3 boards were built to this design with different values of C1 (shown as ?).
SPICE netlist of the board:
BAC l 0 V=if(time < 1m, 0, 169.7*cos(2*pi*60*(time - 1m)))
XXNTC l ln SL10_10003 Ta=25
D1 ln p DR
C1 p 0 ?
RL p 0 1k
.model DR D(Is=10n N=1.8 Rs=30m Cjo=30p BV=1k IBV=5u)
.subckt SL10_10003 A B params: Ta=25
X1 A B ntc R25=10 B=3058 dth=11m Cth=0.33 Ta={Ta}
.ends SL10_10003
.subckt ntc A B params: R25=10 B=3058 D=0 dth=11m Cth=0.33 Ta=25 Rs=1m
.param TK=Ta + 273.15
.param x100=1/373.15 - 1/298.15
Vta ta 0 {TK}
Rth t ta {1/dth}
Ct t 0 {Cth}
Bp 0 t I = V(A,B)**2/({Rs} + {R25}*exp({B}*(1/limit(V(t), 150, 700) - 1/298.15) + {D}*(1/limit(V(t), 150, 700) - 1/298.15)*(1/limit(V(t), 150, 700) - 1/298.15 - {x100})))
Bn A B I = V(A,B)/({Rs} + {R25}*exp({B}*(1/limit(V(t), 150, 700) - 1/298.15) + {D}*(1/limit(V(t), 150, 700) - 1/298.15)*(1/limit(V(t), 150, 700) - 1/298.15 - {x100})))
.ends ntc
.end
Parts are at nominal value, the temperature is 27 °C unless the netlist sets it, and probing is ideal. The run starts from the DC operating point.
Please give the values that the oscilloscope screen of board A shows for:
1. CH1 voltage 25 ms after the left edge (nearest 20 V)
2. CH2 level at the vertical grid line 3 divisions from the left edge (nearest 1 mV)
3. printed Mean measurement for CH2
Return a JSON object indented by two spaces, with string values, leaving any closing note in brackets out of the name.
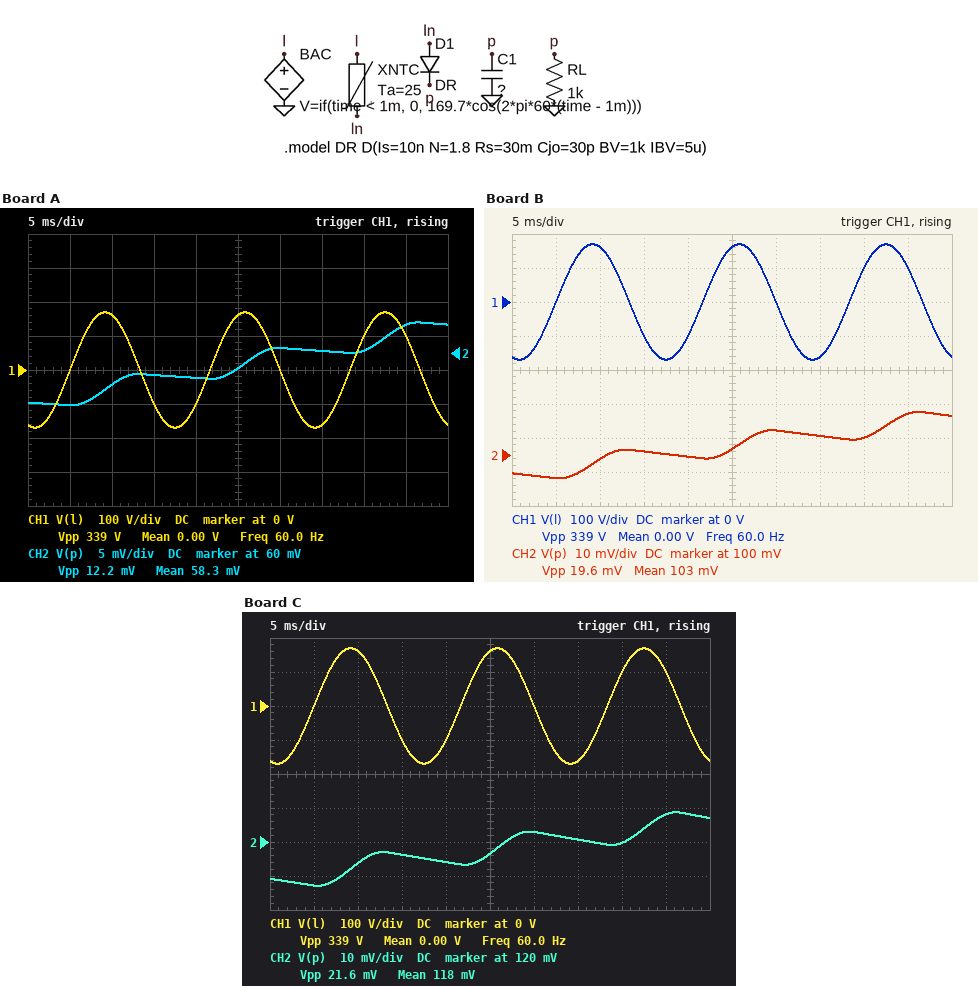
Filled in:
{
  "CH1 voltage 25 ms after the left edge": "160 V",
  "CH2 level at the vertical grid line 3 divisions from the left edge": "57 mV",
  "printed Mean measurement for CH2": "58.3 mV"
}
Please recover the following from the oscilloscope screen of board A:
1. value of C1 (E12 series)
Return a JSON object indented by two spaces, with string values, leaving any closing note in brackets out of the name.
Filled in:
{
  "value of C1": "680 µF"
}
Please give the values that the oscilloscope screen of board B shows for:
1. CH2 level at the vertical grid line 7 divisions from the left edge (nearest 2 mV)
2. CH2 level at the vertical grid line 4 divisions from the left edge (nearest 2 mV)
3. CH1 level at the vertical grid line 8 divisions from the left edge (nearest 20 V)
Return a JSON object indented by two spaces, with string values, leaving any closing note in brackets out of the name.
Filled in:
{
  "CH2 level at the vertical grid line 7 divisions from the left edge": "106 mV",
  "CH2 level at the vertical grid line 4 divisions from the left edge": "100 mV",
  "CH1 level at the vertical grid line 8 divisions from the left edge": "100 V"
}
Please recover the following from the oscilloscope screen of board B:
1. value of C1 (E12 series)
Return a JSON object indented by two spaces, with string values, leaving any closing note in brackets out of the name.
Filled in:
{
  "value of C1": "330 µF"
}
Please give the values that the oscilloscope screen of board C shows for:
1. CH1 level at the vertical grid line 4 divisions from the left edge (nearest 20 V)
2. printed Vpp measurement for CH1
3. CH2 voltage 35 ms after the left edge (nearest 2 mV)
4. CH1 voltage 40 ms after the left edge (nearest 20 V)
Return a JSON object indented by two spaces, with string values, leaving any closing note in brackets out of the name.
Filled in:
{
  "CH1 level at the vertical grid line 4 divisions from the left edge": "-100 V",
  "printed Vpp measurement for CH1": "339 V",
  "CH2 voltage 35 ms after the left edge": "120 mV",
  "CH1 voltage 40 ms after the left edge": "100 V"
}
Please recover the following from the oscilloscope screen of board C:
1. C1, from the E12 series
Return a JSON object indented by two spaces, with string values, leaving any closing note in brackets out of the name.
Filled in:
{
  "C1, from the E12 series": "270 µF"
}
